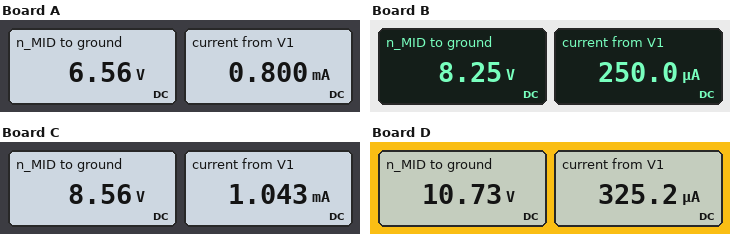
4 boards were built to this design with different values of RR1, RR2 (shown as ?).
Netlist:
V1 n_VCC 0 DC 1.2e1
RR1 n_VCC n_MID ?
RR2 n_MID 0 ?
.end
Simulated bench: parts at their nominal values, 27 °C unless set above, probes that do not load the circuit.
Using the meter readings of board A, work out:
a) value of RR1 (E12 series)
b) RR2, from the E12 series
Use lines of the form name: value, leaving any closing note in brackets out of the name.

value of RR1: 6.8 kΩ
RR2, from the E12 series: 8.2 kΩ
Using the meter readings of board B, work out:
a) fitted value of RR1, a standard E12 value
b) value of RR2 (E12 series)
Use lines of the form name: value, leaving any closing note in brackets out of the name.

fitted value of RR1, a standard E12 value: 15 kΩ
value of RR2: 33 kΩ
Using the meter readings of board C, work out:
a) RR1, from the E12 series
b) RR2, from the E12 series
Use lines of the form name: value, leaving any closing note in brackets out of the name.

RR1, from the E12 series: 3.3 kΩ
RR2, from the E12 series: 8.2 kΩ
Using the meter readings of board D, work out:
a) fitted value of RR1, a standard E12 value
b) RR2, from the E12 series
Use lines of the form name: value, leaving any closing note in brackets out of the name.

fitted value of RR1, a standard E12 value: 3.9 kΩ
RR2, from the E12 series: 33 kΩ
